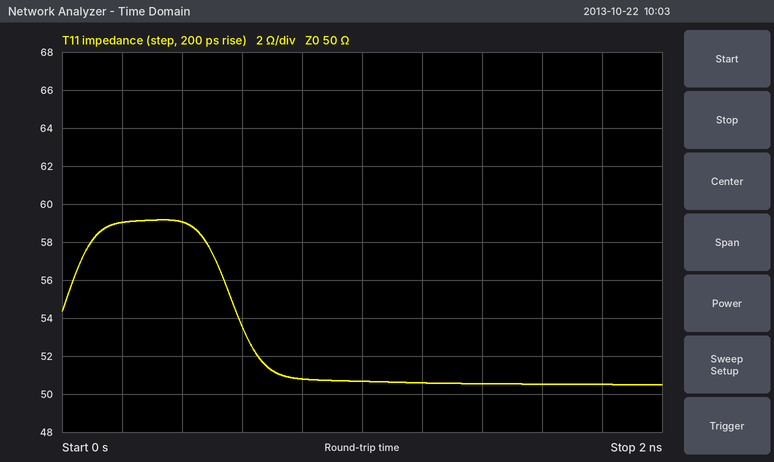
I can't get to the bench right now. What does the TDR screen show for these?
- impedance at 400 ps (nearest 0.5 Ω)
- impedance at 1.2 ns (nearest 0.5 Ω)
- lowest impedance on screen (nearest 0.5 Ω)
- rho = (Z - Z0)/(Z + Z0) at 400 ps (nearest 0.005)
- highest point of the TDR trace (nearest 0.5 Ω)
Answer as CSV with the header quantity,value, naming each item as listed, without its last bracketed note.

quantity,value
impedance at 400 ps,59.0 Ω
impedance at 1.2 ns,50.5 Ω
lowest impedance on screen,50.5 Ω
rho = (Z - Z0)/(Z + Z0) at 400 ps,+0.085
highest point of the TDR trace,59.0 Ω
